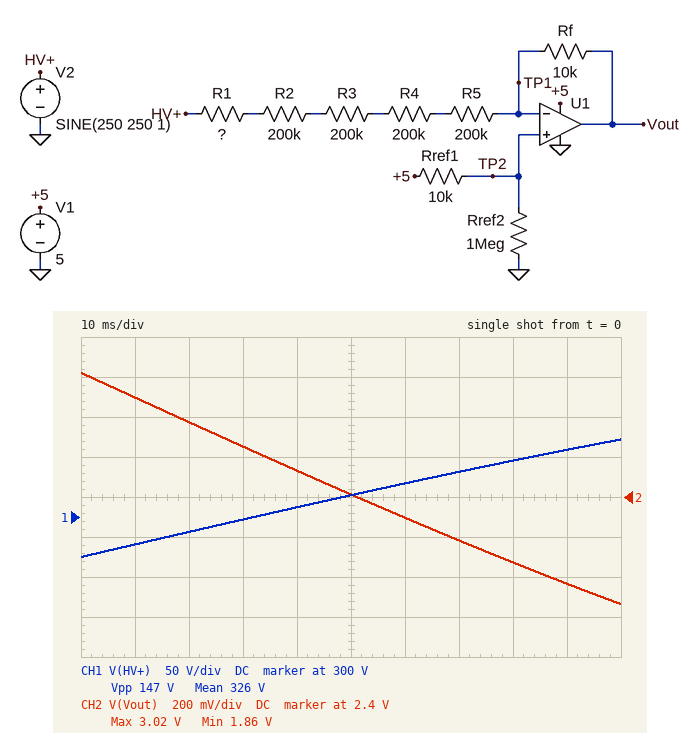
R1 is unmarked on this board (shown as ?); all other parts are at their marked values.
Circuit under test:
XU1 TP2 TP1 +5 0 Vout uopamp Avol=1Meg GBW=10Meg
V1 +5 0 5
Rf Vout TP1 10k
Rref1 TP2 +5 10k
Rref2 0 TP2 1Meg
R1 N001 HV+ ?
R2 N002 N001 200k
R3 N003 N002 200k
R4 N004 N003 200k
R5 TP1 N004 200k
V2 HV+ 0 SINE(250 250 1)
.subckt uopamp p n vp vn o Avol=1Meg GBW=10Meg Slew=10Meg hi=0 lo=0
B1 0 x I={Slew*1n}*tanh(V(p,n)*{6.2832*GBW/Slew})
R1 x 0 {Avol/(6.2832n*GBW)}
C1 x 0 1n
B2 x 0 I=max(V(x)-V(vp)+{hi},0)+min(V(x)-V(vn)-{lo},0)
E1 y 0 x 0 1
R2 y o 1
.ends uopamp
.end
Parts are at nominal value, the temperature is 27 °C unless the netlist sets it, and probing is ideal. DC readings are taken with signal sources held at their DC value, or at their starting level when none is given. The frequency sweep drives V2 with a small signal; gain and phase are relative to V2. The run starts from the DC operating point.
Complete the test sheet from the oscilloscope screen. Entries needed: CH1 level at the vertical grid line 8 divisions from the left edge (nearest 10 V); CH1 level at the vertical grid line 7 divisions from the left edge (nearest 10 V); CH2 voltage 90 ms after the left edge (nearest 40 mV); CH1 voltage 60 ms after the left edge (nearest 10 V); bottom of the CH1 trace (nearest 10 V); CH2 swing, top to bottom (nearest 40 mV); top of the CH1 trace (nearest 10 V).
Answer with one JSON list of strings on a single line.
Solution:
["370 V", "360 V", "1.96 V", "340 V", "250 V", "1.16 V", "400 V"]
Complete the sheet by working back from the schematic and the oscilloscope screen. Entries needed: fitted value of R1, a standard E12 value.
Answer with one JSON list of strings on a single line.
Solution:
["470 kΩ"]
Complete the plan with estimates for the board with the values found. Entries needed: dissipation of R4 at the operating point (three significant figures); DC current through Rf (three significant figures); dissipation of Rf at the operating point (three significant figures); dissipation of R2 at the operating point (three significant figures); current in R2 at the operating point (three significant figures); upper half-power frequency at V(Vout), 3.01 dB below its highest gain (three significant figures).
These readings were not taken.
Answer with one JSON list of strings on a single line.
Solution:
["7.45 mW", "193 µA", "372 µW", "7.45 mW", "193 µA", "9.92 MHz"]
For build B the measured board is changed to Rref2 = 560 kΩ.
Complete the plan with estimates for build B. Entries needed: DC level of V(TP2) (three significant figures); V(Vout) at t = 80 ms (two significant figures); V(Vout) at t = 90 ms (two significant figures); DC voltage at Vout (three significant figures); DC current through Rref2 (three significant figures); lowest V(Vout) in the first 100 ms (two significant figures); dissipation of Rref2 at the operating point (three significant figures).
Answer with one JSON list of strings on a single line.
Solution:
["4.91 V", "2.0 V", "1.9 V", "2.98 V", "8.77 µA", "1.8 V", "43.1 µW"]
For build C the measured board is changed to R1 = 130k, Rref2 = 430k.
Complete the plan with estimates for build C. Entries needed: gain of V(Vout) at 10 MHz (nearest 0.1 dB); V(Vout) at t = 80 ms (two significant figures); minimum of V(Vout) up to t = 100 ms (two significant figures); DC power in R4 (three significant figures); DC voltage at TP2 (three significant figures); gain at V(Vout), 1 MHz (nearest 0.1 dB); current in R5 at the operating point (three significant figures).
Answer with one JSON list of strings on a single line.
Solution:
["-42.4 dB", "960 mV", "670 mV", "13.9 mW", "4.89 V", "-39.4 dB", "264 µA"]
